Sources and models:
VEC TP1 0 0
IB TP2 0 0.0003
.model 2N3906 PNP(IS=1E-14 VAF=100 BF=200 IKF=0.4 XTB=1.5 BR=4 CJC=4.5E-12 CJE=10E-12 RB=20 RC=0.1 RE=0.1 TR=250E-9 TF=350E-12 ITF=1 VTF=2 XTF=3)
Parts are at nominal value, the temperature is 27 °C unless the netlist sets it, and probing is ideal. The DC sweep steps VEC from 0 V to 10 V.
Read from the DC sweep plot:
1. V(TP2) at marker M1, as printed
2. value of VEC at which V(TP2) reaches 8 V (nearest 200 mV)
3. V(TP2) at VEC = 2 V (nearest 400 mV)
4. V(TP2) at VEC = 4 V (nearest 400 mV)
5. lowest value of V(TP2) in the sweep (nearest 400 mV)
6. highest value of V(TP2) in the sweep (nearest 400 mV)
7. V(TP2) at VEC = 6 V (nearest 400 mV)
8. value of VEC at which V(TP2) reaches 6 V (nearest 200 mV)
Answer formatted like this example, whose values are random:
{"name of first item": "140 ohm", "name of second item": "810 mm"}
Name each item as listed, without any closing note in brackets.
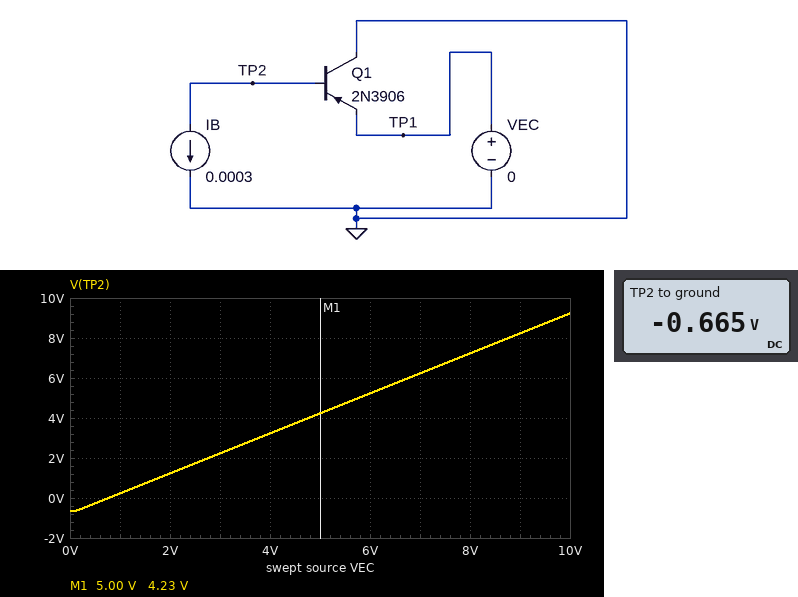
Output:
{"V(TP2) at marker M1, as printed": "4.23 V", "value of VEC at which V(TP2) reaches 8 V": "8.8 V", "V(TP2) at VEC = 2 V": "1.2 V", "V(TP2) at VEC = 4 V": "3.2 V", "lowest value of V(TP2) in the sweep": "-800 mV", "highest value of V(TP2) in the sweep": "9.2 V", "V(TP2) at VEC = 6 V": "5.2 V", "value of VEC at which V(TP2) reaches 6 V": "6.8 V"}
